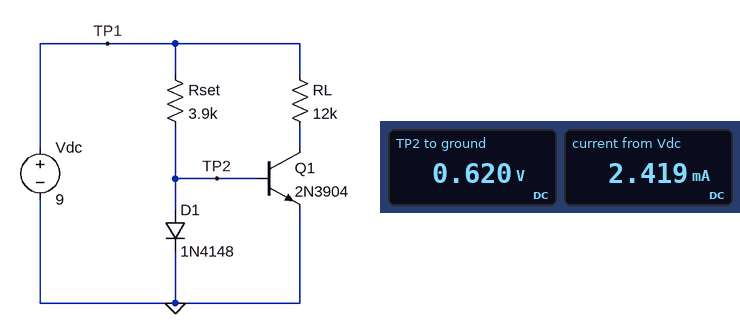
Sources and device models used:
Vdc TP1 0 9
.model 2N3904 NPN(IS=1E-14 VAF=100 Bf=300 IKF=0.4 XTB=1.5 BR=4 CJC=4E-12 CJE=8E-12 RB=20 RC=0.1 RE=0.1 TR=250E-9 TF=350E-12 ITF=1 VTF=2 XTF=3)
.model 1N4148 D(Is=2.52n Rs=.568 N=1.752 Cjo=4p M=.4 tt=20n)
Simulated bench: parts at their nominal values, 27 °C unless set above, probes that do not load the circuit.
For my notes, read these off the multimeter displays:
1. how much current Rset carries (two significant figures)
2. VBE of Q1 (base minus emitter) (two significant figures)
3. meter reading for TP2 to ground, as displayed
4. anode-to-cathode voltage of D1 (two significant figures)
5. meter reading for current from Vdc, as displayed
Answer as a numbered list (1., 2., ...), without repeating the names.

1. 2.1 mA
2. 620 mV
3. 0.620 V
4. 620 mV
5. 2.419 mA
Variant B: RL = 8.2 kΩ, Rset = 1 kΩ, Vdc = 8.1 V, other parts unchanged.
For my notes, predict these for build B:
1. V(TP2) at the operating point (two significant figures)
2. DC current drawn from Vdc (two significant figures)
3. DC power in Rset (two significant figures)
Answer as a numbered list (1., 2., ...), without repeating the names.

1. 680 mV
2. 8.4 mA
3. 55 mW
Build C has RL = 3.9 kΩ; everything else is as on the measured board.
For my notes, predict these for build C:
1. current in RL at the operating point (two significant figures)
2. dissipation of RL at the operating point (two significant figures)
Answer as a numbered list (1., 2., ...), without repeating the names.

1. 280 µA
2. 300 µW
